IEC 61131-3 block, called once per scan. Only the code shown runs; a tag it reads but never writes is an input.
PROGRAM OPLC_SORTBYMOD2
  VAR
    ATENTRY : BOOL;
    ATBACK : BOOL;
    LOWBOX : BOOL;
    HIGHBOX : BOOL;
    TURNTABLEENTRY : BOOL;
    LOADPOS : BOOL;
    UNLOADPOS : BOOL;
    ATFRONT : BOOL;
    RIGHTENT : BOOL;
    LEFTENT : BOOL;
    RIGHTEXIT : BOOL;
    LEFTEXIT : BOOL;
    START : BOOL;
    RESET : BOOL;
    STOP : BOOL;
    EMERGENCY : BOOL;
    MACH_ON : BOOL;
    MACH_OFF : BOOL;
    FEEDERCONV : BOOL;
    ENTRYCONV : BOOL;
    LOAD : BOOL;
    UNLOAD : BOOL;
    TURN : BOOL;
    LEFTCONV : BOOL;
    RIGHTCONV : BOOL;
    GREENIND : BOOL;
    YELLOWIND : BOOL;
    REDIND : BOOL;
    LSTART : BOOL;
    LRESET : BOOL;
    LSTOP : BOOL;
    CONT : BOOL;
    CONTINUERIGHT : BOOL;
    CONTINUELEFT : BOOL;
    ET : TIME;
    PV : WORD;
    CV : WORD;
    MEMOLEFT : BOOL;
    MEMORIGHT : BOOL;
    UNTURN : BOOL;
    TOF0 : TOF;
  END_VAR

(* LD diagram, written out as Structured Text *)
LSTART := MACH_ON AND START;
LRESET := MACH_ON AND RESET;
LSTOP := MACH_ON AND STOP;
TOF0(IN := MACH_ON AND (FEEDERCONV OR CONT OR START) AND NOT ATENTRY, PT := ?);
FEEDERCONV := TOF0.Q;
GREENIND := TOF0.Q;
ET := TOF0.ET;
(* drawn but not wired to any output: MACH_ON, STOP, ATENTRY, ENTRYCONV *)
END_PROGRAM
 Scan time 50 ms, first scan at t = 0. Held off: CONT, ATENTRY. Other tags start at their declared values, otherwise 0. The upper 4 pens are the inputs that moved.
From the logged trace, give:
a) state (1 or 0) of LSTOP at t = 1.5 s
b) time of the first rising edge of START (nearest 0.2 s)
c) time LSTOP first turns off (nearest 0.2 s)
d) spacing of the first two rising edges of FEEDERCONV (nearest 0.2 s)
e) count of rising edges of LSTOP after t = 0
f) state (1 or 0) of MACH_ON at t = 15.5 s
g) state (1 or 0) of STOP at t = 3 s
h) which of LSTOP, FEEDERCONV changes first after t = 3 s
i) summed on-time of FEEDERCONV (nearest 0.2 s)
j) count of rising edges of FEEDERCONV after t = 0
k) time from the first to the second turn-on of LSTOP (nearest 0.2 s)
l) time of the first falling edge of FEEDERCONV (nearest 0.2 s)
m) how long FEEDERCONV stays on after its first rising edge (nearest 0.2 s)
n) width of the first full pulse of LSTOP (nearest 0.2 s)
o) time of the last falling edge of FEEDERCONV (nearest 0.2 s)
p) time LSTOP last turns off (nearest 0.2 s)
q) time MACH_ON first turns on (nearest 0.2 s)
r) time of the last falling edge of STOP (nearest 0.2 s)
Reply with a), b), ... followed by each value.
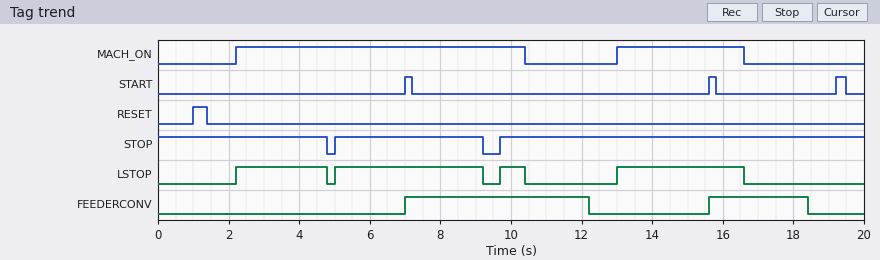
a) 0
b) 7.0 s
c) 4.8 s
d) 8.6 s
e) 4
f) 1
g) 1
h) LSTOP
i) 8.0 s
j) 2
k) 2.8 s
l) 12.2 s
m) 5.2 s
n) 2.6 s
o) 18.4 s
p) 16.6 s
q) 2.2 s
r) 9.2 s
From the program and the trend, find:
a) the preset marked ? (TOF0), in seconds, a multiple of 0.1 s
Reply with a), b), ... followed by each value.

a) 1.8 s
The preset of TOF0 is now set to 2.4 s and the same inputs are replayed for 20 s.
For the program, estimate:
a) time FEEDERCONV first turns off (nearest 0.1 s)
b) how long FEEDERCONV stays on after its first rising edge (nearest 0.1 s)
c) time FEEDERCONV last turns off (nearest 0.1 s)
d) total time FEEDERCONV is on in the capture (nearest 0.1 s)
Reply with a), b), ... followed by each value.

a) 12.8 s
b) 5.8 s
c) 19.0 s
d) 9.2 s
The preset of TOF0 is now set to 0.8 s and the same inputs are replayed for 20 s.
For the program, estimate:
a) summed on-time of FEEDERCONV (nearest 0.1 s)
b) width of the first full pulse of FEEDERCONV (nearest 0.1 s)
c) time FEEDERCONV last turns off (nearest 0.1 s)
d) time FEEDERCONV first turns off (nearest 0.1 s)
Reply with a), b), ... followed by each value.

a) 6.0 s
b) 4.2 s
c) 17.4 s
d) 11.2 s
